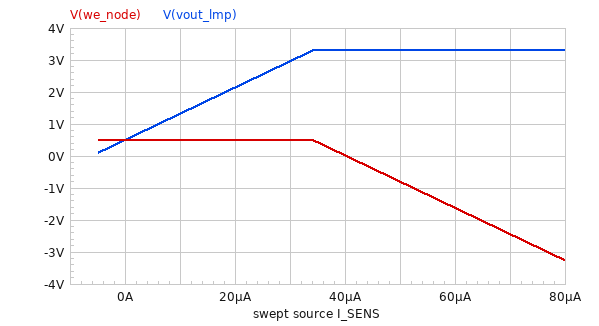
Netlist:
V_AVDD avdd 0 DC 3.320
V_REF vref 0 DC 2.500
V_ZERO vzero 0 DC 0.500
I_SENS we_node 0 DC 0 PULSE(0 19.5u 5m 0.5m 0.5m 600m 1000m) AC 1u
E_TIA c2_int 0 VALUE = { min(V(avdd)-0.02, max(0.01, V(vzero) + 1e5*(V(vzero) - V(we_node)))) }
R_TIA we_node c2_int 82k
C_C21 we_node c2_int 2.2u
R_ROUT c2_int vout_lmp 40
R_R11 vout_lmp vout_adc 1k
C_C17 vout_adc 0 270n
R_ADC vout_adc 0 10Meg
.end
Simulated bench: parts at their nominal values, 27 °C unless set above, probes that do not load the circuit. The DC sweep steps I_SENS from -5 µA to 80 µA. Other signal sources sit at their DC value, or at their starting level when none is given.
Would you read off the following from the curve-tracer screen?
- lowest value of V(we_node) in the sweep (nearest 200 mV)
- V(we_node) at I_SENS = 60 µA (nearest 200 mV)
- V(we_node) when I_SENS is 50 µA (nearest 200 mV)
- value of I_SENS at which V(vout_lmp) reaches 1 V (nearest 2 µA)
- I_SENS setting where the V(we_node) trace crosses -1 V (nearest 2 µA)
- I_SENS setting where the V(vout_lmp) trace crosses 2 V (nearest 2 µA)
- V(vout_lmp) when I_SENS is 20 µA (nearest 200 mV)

-3.2 V
-1.6 V
-800 mV
6 µA
52 µA
18 µA
2.2 V
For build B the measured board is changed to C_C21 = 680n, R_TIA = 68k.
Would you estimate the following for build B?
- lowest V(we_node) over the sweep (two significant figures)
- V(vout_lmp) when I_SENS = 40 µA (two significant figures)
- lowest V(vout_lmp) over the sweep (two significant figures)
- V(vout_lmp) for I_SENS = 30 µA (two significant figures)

-2.1 V
3.2 V
160 mV
2.5 V
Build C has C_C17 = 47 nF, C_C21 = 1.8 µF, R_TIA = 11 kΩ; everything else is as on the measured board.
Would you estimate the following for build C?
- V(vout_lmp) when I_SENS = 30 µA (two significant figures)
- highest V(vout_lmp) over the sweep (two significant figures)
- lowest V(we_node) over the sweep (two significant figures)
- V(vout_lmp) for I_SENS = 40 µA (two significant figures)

830 mV
1.4 V
500 mV
940 mV
